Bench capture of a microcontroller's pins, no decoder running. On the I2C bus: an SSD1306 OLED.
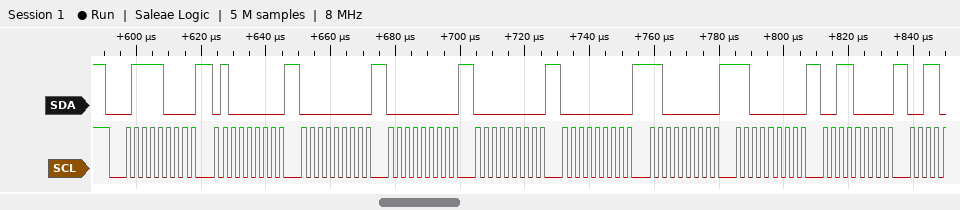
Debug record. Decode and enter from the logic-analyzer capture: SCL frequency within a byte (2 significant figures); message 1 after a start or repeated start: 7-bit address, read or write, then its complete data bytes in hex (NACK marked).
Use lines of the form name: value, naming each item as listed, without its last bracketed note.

SCL frequency within a byte: 400 kHz
message 1 after a start or repeated start: 7-bit address, read or write, then its complete data bytes in hex: 0x3C write: 40 00 00 00 00 C0 C0 30
